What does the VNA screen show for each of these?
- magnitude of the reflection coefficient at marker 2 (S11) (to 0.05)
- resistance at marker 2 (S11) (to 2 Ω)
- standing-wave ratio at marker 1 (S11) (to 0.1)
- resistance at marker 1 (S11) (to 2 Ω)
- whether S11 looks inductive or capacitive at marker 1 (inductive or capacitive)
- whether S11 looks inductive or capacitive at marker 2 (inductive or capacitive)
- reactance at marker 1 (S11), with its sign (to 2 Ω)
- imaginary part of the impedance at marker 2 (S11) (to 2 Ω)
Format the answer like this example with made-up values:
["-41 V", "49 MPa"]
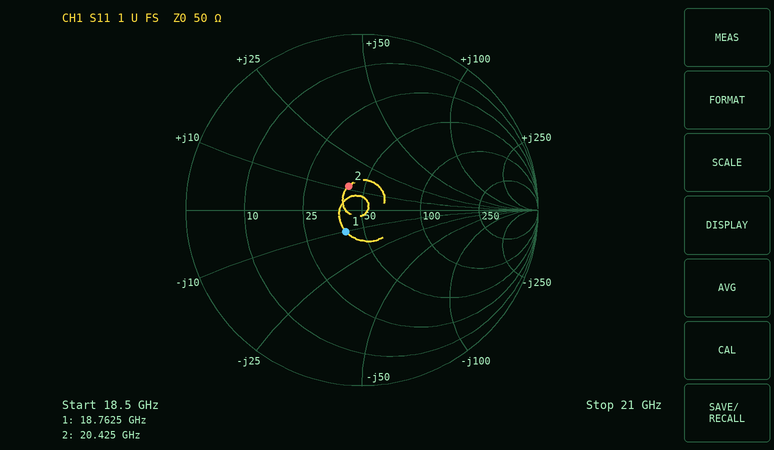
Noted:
["0.15", "42 Ω", "1.4", "40 Ω", "capacitive", "inductive", "-10 Ω", "+12 Ω"]
